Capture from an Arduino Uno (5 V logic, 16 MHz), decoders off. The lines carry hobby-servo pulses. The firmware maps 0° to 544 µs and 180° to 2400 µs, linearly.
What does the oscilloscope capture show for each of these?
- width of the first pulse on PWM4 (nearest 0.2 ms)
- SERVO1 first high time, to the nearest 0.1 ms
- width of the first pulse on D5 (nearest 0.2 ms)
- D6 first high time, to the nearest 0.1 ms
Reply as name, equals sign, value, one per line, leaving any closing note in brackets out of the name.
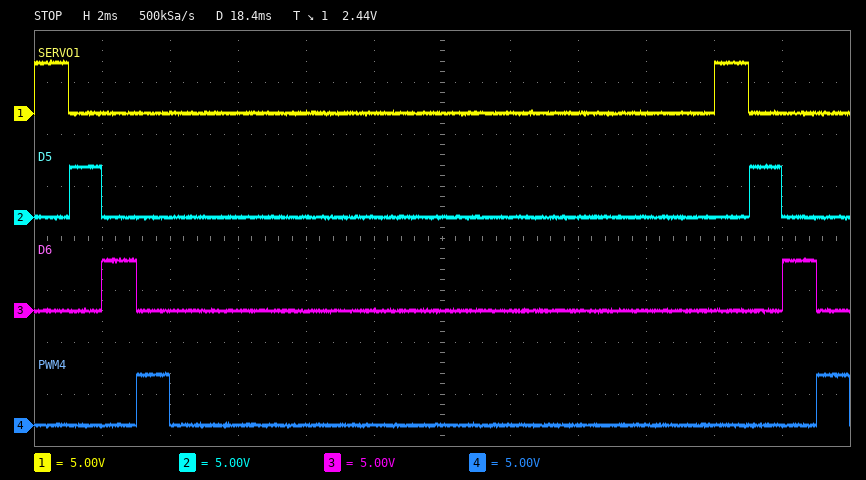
width of the first pulse on PWM4 = 1.0 ms
SERVO1 first high time, to the nearest 0.1 ms = 1.0 ms
width of the first pulse on D5 = 1.0 ms
D6 first high time, to the nearest 0.1 ms = 1.0 ms
